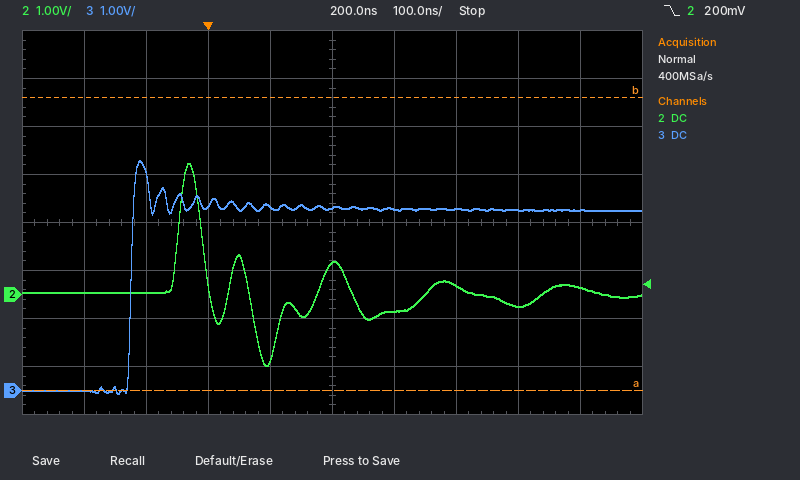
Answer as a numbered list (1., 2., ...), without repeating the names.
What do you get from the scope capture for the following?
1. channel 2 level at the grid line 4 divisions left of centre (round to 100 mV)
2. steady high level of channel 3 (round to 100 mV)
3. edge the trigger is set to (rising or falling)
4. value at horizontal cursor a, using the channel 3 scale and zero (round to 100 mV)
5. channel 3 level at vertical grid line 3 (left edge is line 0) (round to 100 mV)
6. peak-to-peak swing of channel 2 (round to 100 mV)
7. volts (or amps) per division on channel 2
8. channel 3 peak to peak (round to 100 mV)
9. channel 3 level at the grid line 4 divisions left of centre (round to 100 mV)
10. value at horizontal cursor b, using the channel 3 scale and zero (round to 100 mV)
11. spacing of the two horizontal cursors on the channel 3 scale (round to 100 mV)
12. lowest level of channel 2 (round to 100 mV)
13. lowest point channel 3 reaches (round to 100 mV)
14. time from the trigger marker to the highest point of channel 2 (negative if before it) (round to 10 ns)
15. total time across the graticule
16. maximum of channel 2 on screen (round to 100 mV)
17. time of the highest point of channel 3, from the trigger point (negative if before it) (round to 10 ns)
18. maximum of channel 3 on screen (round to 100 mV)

1. 0.0 V
2. 3.8 V
3. falling
4. 0.0 V
5. 3.9 V
6. 4.2 V
7. 1 V
8. 4.9 V
9. 0.0 V
10. 6.1 V
11. 6.1 V
12. -1.5 V
13. -100 mV
14. -30 ns
15. 1 µs
16. 2.7 V
17. -110 ns
18. 4.8 V
